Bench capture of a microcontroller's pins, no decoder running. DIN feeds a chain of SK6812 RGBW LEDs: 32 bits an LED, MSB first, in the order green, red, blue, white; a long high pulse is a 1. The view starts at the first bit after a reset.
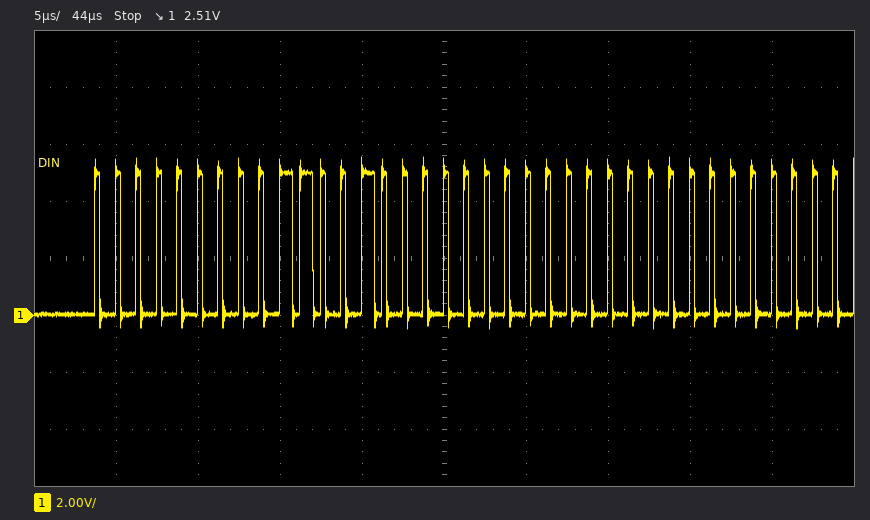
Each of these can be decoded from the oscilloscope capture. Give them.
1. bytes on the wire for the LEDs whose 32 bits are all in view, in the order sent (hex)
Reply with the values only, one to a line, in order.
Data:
00 64 00 00
